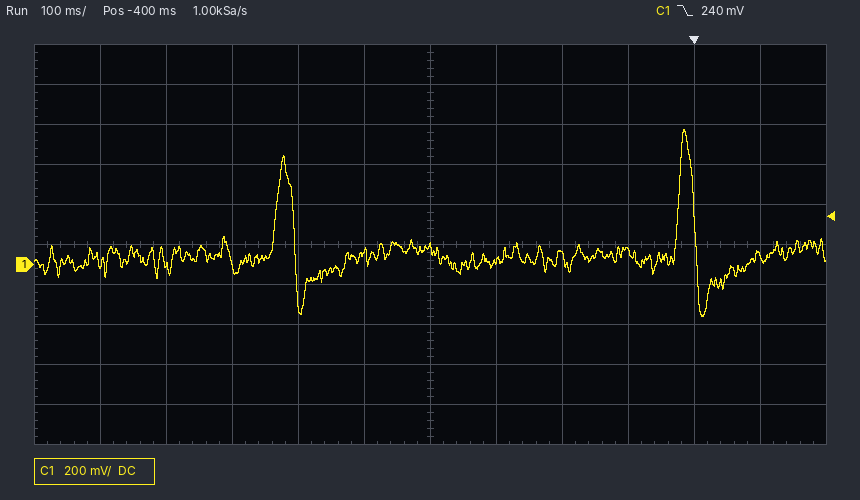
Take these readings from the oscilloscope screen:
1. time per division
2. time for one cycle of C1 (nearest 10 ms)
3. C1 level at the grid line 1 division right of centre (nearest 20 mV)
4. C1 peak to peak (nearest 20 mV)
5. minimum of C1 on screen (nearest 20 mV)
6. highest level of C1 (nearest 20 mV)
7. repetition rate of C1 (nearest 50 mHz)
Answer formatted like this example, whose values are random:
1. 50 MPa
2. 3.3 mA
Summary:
1. 100 ms
2. 610 ms
3. 20 mV
4. 940 mV
5. -260 mV
6. 680 mV
7. 1.65 Hz
